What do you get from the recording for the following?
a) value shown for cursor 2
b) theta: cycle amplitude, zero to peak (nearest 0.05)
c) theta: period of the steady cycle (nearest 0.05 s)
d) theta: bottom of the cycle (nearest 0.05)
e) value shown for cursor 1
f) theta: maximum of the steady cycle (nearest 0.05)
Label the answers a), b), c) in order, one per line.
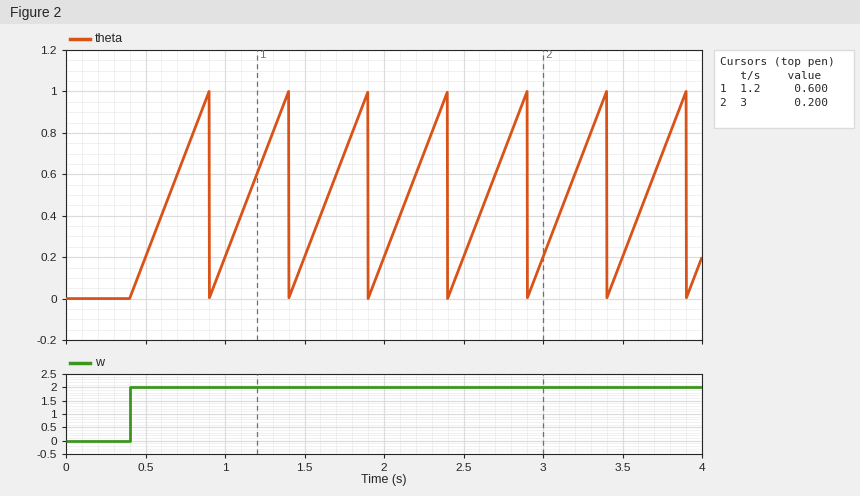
a) 0.200
b) 0.50
c) 0.50 s
d) 0.00
e) 0.600
f) 1.00
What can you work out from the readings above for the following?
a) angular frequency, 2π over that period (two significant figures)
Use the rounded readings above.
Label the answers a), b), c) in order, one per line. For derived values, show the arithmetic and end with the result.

a) 2π / 0.5 = 13 rad/s
